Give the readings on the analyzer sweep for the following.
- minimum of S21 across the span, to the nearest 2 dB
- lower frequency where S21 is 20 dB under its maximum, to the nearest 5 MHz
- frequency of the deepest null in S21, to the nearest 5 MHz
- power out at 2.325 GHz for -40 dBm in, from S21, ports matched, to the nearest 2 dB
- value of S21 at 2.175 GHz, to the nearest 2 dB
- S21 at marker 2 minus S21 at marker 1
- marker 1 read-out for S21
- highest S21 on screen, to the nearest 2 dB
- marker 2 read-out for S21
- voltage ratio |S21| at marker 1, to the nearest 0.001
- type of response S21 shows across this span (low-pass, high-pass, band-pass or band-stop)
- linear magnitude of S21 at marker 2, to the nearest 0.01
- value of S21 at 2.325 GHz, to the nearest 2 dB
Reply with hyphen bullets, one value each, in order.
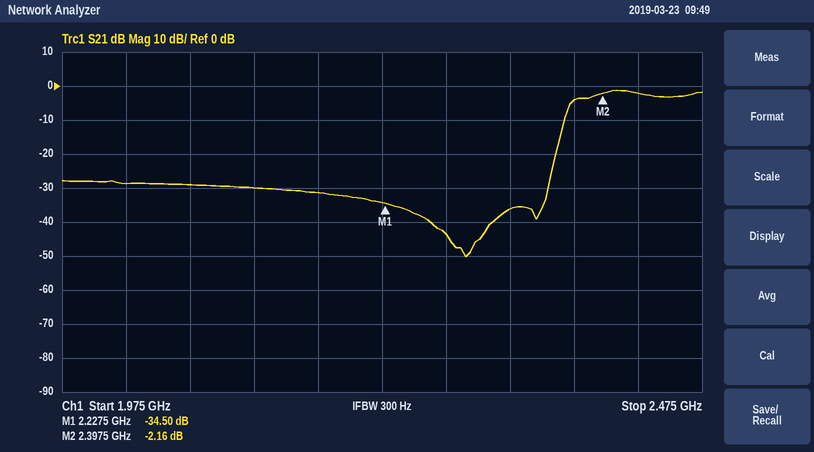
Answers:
- -50 dB
- 2.360 GHz
- 2.290 GHz
- -76 dBm
- -32 dB
- 32.34 dB
- -34.50 dB
- -2 dB
- -2.16 dB
- 0.019
- high-pass
- 0.78
- -36 dB
